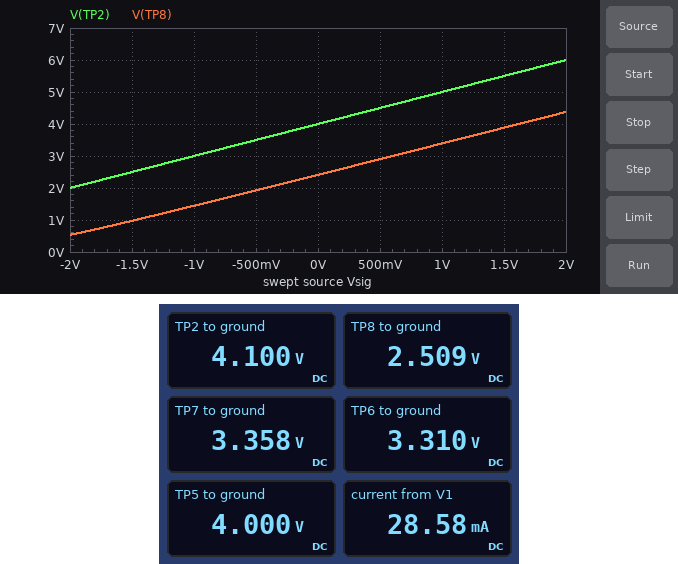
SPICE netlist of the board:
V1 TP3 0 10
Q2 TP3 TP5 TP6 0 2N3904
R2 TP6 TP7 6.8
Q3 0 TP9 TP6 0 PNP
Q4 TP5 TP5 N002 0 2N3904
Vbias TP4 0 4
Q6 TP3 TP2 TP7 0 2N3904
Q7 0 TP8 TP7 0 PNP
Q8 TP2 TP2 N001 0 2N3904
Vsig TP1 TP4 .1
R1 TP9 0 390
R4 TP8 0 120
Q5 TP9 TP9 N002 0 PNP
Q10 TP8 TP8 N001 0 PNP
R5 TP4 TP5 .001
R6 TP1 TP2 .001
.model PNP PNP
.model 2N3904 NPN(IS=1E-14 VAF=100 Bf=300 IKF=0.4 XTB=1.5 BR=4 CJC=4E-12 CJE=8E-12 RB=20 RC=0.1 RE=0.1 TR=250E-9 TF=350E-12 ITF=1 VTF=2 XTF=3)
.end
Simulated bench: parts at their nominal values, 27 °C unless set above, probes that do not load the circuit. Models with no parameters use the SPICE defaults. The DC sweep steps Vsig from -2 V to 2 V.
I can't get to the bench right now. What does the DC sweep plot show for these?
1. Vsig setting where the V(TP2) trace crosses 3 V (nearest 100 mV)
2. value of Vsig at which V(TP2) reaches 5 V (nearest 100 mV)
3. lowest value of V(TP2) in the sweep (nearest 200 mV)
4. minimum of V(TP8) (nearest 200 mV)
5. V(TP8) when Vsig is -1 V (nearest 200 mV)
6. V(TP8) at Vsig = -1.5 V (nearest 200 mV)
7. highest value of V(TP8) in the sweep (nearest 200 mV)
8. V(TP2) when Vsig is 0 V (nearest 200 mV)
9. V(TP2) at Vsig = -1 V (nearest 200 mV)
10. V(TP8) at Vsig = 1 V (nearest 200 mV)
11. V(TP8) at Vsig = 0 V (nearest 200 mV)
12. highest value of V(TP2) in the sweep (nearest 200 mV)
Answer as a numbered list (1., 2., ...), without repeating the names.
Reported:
1. -1.0 V
2. 1.0 V
3. 2.0 V
4. 600 mV
5. 1.4 V
6. 1.0 V
7. 4.4 V
8. 4.0 V
9. 3.0 V
10. 3.4 V
11. 2.4 V
12. 6.0 V
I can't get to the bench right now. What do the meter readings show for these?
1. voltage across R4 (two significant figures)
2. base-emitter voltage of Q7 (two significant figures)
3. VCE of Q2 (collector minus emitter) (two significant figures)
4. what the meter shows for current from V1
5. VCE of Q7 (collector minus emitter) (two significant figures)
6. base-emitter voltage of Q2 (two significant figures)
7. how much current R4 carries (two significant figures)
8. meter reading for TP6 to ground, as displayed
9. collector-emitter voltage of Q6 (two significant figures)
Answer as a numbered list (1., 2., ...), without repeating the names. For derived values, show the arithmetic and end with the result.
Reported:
1. 2.509 V = 2.5 V
2. 2.509 V - 3.358 V = -850 mV
3. 10 V - 3.31 V = 6.7 V
4. 28.58 mA
5. 0 V - 3.358 V = -3.4 V
6. 4 V - 3.31 V = 690 mV
7. (2.509 V) / 120 Ω = 21 mA
8. 3.310 V
9. 10 V - 3.358 V = 6.6 V
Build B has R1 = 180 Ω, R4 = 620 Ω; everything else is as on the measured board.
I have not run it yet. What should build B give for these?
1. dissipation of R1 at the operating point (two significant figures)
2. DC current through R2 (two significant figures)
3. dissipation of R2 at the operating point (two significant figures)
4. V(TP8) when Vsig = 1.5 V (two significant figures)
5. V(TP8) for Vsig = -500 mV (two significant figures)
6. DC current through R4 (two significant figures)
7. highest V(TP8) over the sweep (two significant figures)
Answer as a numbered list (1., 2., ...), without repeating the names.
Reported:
1. 33 mW
2. 13 mA
3. 1.1 mW
4. 4.0 V
5. 2.0 V
6. 4.2 mA
7. 4.5 V
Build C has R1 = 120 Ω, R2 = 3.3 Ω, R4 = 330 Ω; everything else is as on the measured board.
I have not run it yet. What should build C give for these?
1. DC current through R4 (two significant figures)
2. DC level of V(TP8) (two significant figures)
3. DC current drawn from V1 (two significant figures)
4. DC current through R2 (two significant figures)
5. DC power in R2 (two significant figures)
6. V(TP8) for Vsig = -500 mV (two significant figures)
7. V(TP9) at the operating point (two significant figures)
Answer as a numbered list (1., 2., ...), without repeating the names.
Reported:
1. 7.8 mA
2. 2.6 V
3. 38 mA
4. 24 mA
5. 1.8 mW
6. 2.0 V
7. 2.4 V
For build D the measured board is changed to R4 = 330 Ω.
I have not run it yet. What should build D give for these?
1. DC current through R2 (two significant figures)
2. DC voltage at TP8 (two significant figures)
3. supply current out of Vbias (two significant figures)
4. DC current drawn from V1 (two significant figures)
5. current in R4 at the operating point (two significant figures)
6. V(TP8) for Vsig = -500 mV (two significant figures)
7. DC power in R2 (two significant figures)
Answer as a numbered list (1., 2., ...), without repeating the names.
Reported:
1. 9.1 mA
2. 2.6 V
3. 14 mA
4. 17 mA
5. 7.8 mA
6. 2.0 V
7. 560 µW
